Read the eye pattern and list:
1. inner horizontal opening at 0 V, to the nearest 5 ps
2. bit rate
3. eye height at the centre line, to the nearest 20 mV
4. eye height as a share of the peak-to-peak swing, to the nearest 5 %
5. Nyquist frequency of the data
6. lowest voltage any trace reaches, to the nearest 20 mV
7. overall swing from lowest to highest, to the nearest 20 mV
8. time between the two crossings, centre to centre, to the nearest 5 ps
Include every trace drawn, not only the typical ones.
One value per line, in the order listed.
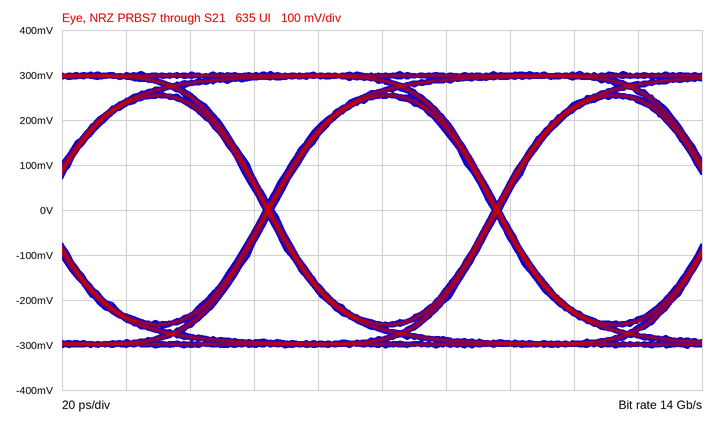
70 ps
14 Gb/s
500 mV
80 %
7 GHz
-300 mV
620 mV
70 ps
